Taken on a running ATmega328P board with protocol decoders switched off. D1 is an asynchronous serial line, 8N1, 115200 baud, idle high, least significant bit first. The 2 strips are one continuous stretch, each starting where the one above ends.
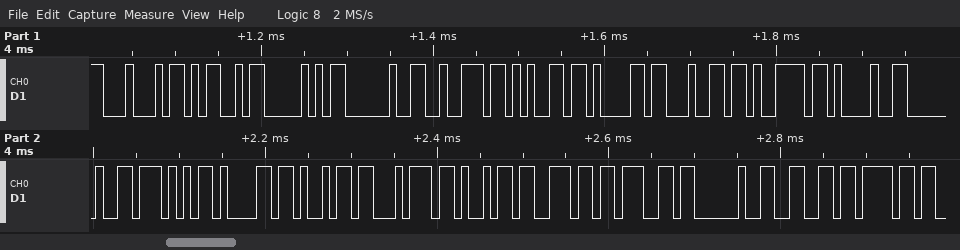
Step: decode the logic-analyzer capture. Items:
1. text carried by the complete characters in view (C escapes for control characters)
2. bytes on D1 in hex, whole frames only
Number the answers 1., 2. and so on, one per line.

1. "DMP ready! Waiting fo"
2. 0x44 0x4D 0x50 0x20 0x72 0x65 0x61 0x64 0x79 0x21 0x20 0x57 0x61 0x69 0x74 0x69 0x6E 0x67 0x20 0x66 0x6F
